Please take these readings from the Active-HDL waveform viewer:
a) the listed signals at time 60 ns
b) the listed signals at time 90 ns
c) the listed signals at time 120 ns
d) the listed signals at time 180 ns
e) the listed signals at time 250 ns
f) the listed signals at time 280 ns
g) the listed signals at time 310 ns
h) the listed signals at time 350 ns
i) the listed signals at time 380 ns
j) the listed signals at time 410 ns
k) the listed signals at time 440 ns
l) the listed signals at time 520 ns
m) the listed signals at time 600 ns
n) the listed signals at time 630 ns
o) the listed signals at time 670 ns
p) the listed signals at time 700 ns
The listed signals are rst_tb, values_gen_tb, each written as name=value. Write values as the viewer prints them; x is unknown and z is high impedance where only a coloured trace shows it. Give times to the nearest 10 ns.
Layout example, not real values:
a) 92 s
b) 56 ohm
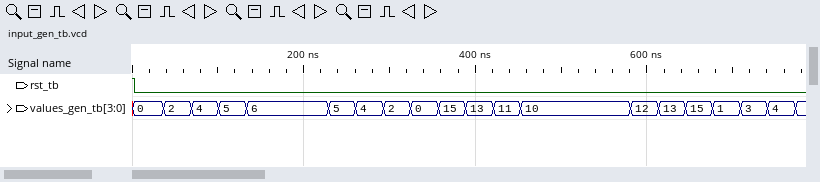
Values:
a) rst_tb=0, values_gen_tb=2
b) rst_tb=0, values_gen_tb=4
c) rst_tb=0, values_gen_tb=5
d) rst_tb=0, values_gen_tb=6
e) rst_tb=0, values_gen_tb=5
f) rst_tb=0, values_gen_tb=4
g) rst_tb=0, values_gen_tb=2
h) rst_tb=0, values_gen_tb=0
i) rst_tb=0, values_gen_tb=15
j) rst_tb=0, values_gen_tb=13
k) rst_tb=0, values_gen_tb=11
l) rst_tb=0, values_gen_tb=10
m) rst_tb=0, values_gen_tb=12
n) rst_tb=0, values_gen_tb=13
o) rst_tb=0, values_gen_tb=15
p) rst_tb=0, values_gen_tb=1
